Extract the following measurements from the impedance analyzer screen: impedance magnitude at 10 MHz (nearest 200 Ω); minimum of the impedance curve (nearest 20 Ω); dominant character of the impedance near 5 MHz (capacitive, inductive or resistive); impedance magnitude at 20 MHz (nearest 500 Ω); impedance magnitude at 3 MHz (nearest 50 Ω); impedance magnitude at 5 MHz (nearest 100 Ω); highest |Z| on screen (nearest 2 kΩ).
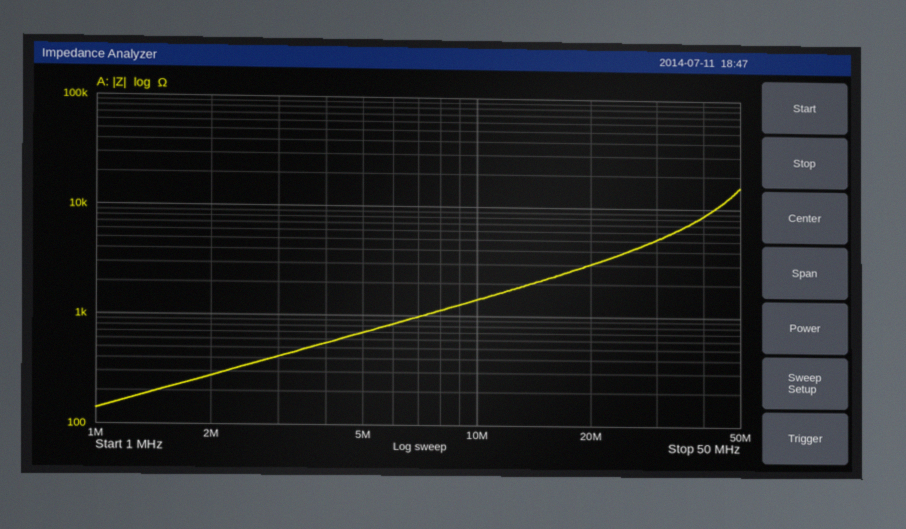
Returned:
1.4 kΩ
140 Ω
inductive
3.0 kΩ
400 Ω
700 Ω
16 kΩ
